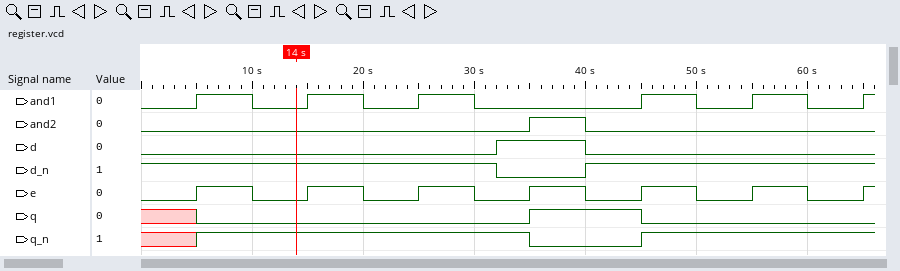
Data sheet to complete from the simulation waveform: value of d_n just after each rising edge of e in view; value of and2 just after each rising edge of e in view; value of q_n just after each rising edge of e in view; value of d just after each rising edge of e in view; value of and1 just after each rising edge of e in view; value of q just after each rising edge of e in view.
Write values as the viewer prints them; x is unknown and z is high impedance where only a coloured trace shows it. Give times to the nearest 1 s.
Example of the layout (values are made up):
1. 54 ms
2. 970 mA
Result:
1. 1 1 1 0 1 1 1
2. 0 0 0 1 0 0 0
3. 1 1 1 0 1 1 1
4. 0 0 0 1 0 0 0
5. 1 1 1 0 1 1 1
6. 0 0 0 1 0 0 0
